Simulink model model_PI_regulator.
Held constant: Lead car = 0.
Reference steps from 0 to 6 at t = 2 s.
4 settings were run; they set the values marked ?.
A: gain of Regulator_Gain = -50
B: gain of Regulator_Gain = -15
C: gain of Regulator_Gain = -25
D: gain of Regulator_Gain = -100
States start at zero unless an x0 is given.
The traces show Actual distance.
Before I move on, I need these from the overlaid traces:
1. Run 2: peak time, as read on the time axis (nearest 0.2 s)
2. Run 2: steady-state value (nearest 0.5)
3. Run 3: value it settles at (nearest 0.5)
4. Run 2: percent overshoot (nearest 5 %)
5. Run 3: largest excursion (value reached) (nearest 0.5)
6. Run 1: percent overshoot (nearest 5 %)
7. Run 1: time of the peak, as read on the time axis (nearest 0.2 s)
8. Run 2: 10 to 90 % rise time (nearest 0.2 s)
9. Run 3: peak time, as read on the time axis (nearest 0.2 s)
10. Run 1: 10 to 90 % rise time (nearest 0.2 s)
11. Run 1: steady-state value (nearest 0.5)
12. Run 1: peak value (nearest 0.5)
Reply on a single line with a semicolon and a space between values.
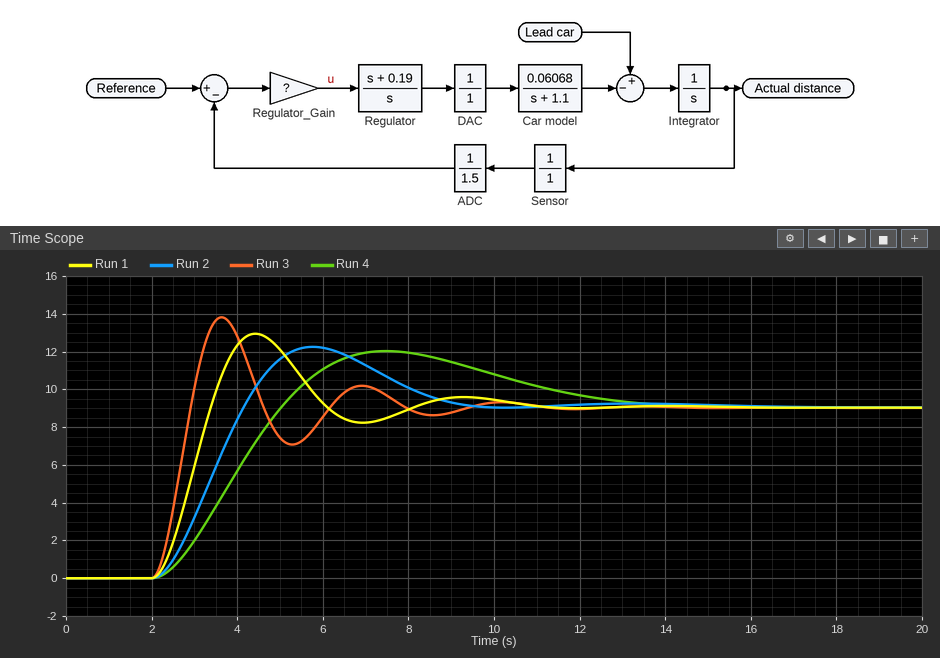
5.8 s; 9.0; 9.0; 35 %; 14.0; 45 %; 4.4 s; 1.4 s; 3.6 s; 1.0 s; 9.0; 13.0
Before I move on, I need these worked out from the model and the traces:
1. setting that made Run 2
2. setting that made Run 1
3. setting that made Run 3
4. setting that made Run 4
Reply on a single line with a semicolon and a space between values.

C; A; D; B
